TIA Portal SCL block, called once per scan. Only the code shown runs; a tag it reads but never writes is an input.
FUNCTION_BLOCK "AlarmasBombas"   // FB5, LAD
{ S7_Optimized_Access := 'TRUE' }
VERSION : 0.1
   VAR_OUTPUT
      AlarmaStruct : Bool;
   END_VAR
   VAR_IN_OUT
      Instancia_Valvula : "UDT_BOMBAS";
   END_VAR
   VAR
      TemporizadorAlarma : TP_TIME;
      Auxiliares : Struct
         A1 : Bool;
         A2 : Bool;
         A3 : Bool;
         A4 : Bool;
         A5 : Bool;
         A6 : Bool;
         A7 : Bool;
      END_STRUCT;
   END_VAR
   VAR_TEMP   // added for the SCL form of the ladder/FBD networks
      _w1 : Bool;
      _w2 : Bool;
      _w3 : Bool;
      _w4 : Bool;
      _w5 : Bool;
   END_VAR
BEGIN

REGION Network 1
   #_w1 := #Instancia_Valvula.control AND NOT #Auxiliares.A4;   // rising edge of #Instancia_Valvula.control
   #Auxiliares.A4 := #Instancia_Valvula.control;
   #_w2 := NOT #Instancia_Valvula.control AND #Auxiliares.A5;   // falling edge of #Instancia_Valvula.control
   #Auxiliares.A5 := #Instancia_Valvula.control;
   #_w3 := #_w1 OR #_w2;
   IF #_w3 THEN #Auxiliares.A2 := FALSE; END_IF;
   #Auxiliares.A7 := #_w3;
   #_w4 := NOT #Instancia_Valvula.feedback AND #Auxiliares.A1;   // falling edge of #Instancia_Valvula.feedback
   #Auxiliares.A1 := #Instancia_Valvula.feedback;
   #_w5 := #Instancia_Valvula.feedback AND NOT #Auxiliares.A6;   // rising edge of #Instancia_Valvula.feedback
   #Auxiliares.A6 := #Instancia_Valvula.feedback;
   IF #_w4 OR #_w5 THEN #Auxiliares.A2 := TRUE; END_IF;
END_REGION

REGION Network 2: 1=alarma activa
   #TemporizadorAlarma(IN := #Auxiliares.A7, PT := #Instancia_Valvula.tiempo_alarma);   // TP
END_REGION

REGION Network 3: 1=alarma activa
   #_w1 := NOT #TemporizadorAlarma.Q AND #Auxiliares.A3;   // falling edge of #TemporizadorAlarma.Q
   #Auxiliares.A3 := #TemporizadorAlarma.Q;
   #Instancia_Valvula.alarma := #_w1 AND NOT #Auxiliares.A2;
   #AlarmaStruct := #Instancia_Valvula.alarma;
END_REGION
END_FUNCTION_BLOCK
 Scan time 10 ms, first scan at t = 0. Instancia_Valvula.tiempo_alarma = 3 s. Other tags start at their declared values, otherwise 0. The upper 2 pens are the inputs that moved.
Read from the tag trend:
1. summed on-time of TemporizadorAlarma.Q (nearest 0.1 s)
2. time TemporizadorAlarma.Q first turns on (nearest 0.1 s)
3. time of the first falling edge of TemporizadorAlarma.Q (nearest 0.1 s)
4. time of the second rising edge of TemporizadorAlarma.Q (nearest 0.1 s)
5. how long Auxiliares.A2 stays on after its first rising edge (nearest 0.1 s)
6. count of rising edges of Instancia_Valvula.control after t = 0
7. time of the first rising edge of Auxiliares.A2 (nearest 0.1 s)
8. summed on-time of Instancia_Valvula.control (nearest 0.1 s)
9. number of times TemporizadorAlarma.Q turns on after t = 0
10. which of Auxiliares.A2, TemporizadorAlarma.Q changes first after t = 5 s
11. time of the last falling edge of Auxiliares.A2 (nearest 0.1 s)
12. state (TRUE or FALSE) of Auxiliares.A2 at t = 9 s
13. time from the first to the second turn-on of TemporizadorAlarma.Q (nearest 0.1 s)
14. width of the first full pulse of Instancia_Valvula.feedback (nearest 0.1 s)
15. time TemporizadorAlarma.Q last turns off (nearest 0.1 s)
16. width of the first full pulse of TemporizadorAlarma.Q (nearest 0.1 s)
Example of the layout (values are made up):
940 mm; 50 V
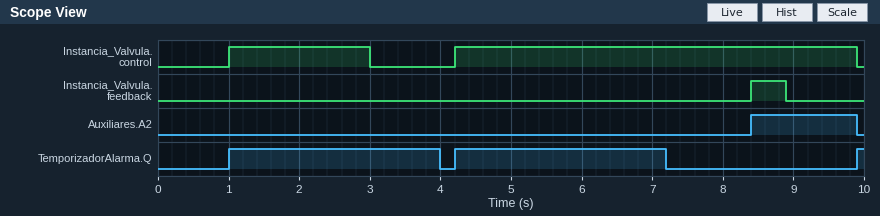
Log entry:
6.1 s; 1.0 s; 4.0 s; 4.2 s; 1.5 s; 2; 8.4 s; 7.7 s; 3; TemporizadorAlarma.Q; 9.9 s; TRUE; 3.2 s; 0.5 s; 7.2 s; 3.0 s
